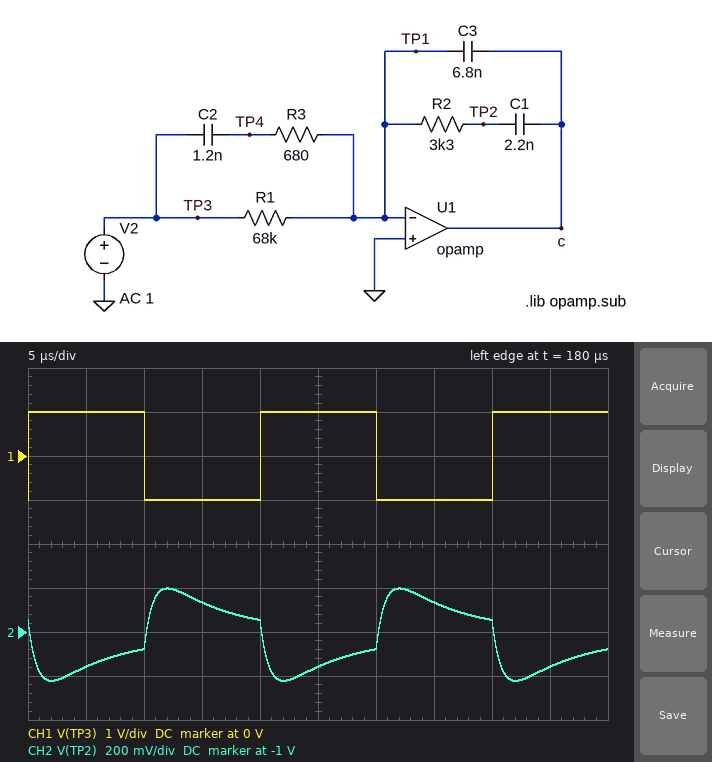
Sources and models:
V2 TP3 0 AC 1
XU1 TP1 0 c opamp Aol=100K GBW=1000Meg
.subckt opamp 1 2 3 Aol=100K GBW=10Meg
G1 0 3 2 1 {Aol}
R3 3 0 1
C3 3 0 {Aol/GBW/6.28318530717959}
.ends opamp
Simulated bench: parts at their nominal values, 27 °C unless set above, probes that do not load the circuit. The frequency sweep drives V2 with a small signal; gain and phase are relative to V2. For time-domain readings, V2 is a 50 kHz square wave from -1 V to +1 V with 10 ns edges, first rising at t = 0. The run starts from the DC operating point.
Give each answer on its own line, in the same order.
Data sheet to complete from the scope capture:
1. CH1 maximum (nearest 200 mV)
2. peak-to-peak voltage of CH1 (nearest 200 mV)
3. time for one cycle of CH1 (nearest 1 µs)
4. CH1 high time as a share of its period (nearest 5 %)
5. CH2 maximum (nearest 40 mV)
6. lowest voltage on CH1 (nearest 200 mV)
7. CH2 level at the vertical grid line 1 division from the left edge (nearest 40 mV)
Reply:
1.0 V
2.0 V
20 µs
50 %
-800 mV
-1.0 V
-1.16 V
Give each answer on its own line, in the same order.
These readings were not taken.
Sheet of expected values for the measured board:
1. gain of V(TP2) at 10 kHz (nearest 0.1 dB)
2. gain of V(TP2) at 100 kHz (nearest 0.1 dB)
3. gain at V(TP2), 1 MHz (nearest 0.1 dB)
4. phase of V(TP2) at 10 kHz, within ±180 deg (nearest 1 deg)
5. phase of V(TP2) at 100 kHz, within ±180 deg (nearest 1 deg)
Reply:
-24.6 dB
-16.3 dB
-29.3 dB
-123 deg
168 deg
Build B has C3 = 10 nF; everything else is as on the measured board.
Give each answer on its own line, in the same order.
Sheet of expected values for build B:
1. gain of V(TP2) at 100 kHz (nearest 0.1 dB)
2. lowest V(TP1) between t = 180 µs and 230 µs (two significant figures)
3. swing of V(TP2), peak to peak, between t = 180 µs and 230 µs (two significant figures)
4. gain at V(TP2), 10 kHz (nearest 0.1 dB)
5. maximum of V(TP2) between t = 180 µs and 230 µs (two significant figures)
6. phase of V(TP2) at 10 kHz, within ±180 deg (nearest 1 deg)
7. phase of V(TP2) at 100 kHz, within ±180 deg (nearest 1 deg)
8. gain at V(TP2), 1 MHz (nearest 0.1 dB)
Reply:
-19.6 dB
-1.0 V
280 mV
-27.3 dB
-870 mV
-124 deg
167 deg
-32.7 dB
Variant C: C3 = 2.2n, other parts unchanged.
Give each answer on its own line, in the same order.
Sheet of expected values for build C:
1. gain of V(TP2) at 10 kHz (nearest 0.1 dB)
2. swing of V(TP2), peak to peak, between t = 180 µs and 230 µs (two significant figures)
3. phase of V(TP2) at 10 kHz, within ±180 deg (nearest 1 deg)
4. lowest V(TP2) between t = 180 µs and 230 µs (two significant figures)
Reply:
-18.1 dB
1.3 V
-117 deg
-1.7 V
